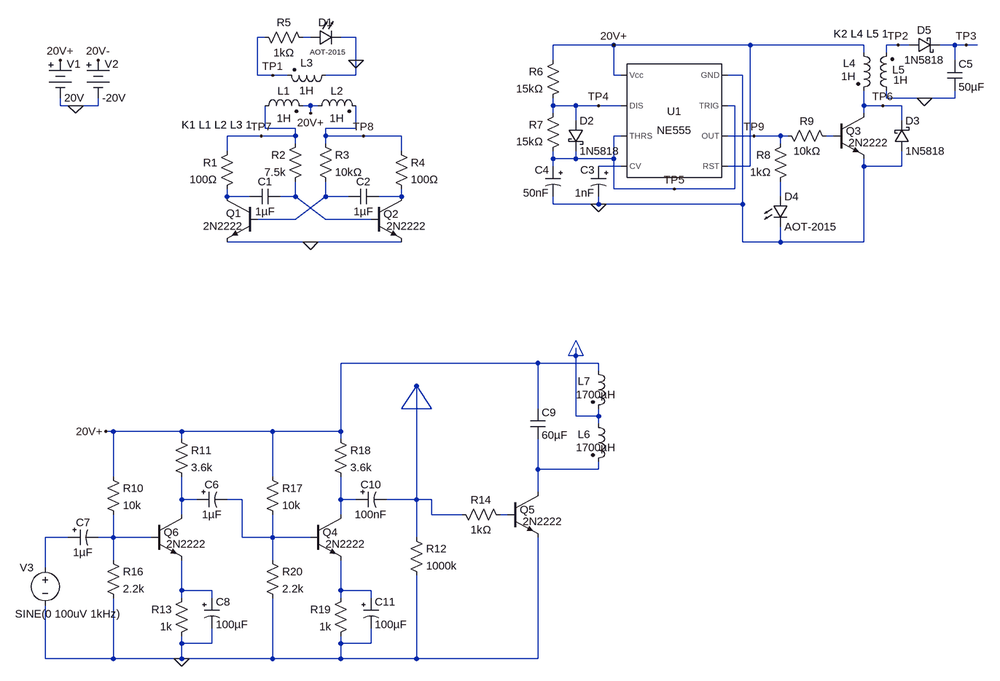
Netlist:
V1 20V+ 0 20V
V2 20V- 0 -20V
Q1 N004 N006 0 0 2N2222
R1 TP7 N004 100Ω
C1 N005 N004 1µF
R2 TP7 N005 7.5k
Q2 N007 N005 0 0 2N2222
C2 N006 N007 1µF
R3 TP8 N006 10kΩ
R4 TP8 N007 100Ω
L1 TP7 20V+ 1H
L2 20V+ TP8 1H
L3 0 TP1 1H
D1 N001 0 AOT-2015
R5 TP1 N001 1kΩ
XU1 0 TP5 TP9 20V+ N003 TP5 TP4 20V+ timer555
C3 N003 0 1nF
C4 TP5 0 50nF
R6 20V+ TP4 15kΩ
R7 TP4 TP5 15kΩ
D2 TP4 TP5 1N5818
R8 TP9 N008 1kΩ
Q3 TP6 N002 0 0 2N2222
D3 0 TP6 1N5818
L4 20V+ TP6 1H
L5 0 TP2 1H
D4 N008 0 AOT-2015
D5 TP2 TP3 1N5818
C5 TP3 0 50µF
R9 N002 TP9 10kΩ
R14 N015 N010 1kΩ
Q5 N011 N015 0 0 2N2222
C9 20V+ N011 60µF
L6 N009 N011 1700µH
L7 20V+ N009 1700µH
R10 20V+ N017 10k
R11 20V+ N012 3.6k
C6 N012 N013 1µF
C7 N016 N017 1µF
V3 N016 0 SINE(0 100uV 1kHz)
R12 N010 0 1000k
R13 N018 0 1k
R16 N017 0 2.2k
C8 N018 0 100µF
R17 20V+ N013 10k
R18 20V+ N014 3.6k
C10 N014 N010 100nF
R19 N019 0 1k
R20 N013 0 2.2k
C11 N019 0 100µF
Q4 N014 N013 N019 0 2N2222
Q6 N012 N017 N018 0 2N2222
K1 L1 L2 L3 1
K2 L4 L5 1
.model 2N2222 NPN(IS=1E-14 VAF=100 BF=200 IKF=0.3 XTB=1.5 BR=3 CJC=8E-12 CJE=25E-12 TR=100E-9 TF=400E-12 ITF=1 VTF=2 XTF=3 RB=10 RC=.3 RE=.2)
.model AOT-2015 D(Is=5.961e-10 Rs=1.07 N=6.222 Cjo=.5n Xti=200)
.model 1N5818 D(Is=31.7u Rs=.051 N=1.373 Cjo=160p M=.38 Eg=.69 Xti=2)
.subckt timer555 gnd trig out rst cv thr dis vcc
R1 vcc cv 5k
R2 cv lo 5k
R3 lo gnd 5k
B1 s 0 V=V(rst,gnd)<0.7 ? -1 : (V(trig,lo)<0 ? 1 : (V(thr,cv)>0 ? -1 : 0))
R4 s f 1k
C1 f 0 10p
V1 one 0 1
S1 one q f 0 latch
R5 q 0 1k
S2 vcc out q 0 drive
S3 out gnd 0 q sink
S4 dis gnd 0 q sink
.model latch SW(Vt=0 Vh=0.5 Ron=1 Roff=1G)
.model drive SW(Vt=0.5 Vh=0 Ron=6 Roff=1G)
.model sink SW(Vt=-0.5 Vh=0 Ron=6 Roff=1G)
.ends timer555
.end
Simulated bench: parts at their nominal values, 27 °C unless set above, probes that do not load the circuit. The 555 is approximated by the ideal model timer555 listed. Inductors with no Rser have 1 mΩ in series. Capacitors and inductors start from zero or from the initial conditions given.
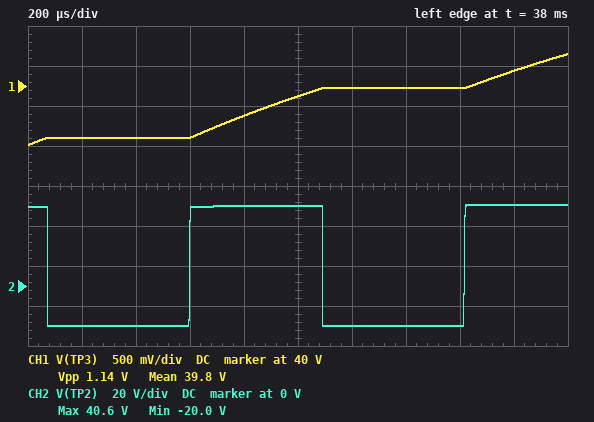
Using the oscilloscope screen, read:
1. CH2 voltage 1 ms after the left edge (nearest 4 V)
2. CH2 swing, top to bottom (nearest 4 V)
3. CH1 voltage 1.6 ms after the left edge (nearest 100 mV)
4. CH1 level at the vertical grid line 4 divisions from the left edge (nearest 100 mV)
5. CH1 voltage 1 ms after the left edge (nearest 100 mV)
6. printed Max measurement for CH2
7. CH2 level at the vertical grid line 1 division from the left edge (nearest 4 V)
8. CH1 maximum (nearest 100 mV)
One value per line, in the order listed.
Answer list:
40 V
60 V
40.0 V
39.6 V
39.9 V
40.6 V
-20 V
40.4 V
